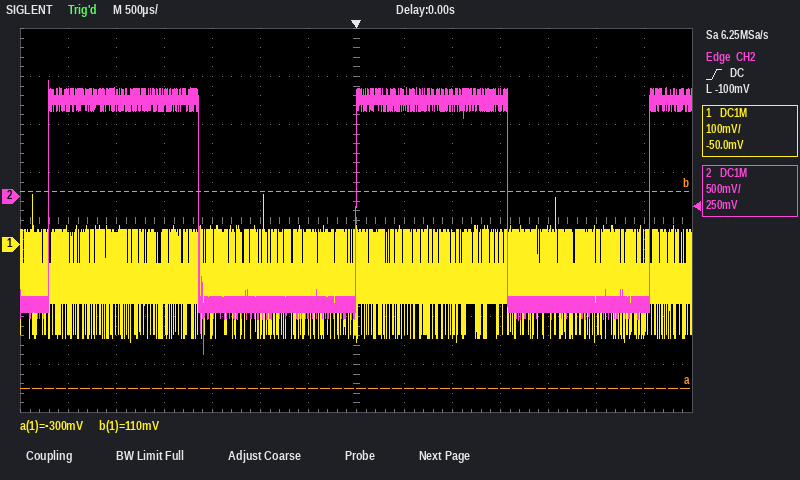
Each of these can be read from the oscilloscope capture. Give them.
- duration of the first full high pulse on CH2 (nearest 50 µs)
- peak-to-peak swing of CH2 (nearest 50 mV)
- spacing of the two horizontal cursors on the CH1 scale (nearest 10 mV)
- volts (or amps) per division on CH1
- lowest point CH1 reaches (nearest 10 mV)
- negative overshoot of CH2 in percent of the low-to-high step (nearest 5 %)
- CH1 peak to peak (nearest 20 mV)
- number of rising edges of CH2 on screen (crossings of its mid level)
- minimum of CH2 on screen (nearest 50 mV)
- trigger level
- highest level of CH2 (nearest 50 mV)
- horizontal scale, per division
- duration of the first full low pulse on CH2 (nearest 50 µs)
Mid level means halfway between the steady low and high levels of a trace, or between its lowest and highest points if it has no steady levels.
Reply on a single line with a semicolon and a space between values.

1.55 ms; 2.85 V; 410 mV; 100 mV; -200 mV; 25 %; 300 mV; 3; -1.65 V; -100 mV; 1.20 V; 500 µs; 1.65 ms
